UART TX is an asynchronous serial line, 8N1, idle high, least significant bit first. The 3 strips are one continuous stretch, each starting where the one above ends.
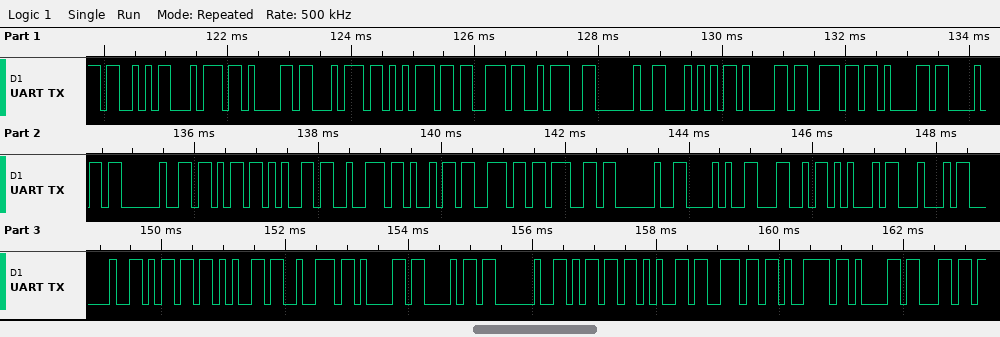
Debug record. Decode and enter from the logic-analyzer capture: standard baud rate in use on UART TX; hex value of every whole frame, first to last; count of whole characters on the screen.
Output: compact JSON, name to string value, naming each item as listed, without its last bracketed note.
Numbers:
{"standard baud rate in use on UART TX": "9600 baud", "hex value of every whole frame, first to last": "0x53 0x74 0x61 0x74 0x75 0x73 0x3A 0x20 0x54 0x61 0x6E 0x61 0x68 0x20 0x6B 0x65 0x72 0x69 0x6E 0x67 0x20 0x28 0x4C 0x45 0x44 0x20 0x6D 0x65 0x72 0x61 0x68 0x20 0x6D 0x65 0x6E 0x79 0x61 0x6C", "count of whole characters on the screen": "38"}
